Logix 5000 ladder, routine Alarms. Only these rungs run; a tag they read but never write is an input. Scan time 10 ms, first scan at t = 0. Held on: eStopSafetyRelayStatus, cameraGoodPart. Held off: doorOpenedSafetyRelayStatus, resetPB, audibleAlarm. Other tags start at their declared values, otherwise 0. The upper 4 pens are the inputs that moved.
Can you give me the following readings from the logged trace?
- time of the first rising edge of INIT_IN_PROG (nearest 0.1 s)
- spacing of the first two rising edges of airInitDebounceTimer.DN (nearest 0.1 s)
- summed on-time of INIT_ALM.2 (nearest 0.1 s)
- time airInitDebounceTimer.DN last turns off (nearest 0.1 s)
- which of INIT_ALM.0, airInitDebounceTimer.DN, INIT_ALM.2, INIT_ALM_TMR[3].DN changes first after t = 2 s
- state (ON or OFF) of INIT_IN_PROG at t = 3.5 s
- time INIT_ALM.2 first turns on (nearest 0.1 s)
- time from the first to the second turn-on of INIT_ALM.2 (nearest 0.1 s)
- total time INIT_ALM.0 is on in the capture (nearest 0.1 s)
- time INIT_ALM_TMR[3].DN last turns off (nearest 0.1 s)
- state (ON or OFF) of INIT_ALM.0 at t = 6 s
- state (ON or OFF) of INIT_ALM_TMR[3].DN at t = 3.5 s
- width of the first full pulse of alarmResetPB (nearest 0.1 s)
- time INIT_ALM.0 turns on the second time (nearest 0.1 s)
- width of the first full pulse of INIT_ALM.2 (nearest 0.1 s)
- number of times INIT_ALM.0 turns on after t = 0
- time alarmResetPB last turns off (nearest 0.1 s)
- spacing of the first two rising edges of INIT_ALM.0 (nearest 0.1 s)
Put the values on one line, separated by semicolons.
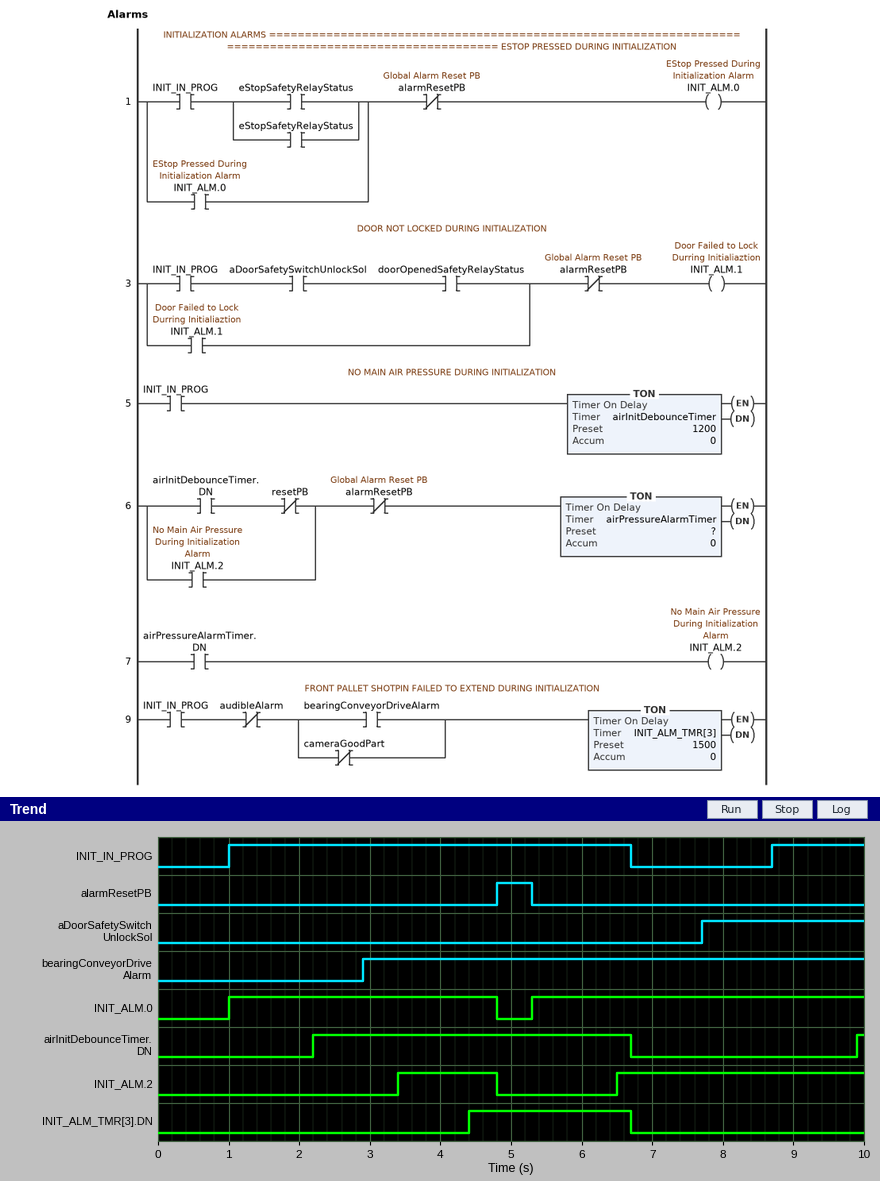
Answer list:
1.0 s; 7.7 s; 4.9 s; 6.7 s; airInitDebounceTimer.DN; ON; 3.4 s; 3.1 s; 8.5 s; 6.7 s; ON; OFF; 0.5 s; 5.3 s; 1.4 s; 2; 5.3 s; 4.3 s
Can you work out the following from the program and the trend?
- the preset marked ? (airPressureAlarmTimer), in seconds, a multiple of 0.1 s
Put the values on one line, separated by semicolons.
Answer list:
1.2 s
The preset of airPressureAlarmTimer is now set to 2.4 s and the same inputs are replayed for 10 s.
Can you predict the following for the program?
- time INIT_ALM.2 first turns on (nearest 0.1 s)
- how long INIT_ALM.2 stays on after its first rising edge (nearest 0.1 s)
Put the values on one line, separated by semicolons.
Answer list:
4.6 s; 0.2 s
